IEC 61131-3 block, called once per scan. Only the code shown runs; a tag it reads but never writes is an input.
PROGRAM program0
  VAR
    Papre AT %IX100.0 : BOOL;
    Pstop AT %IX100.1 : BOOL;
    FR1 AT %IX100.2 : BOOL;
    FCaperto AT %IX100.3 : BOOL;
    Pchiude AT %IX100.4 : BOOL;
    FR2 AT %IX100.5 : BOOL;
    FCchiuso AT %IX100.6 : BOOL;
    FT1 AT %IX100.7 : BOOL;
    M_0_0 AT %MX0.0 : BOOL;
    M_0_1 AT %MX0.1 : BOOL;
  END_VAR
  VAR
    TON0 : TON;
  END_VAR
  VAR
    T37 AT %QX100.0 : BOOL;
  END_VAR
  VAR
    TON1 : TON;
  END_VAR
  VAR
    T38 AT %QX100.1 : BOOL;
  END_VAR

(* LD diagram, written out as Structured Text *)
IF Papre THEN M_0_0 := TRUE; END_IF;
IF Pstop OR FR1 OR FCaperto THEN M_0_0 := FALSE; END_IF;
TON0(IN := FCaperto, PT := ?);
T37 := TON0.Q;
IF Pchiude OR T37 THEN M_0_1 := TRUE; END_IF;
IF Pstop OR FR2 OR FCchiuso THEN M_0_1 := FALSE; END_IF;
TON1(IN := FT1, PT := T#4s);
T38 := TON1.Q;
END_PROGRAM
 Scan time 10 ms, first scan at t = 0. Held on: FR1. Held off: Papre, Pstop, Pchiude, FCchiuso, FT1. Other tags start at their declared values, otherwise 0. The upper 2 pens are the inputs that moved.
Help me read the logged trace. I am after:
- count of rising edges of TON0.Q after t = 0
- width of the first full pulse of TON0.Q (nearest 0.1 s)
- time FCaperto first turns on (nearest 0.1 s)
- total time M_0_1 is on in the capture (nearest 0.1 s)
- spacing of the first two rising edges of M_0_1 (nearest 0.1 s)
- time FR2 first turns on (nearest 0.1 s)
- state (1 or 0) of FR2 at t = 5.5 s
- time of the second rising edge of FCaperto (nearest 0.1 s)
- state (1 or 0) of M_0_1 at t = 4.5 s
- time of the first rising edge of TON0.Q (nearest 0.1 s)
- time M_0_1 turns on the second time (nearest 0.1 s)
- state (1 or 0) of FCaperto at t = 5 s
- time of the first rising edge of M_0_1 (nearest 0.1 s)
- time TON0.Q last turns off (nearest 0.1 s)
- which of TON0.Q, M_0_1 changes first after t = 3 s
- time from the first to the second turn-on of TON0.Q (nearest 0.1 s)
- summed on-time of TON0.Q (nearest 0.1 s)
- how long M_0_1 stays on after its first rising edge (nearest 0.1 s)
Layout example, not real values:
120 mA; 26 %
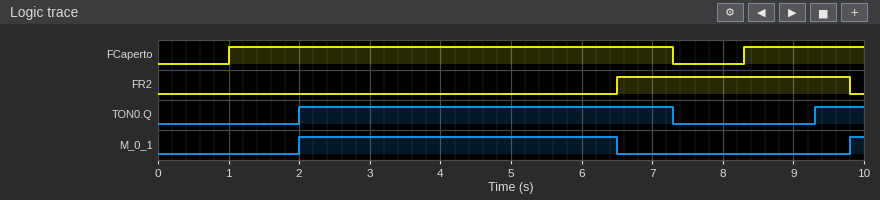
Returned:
2; 5.3 s; 1.0 s; 4.7 s; 7.8 s; 6.5 s; 0; 8.3 s; 1; 2.0 s; 9.8 s; 1; 2.0 s; 7.3 s; M_0_1; 7.3 s; 6.0 s; 4.5 s
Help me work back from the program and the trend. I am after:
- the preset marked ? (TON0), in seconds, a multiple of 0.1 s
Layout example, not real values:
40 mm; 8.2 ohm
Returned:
1.0 s
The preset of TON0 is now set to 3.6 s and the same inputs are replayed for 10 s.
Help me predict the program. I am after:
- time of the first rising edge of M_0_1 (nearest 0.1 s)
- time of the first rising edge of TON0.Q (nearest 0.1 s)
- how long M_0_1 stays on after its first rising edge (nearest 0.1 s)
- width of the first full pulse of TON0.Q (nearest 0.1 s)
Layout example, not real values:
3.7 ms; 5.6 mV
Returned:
4.6 s; 4.6 s; 1.9 s; 2.7 s
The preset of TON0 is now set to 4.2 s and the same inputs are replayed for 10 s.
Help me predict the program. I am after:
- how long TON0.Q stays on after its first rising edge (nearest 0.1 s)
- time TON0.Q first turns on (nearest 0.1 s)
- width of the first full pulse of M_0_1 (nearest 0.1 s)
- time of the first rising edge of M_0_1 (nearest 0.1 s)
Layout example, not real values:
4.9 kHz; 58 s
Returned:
2.1 s; 5.2 s; 1.3 s; 5.2 s
